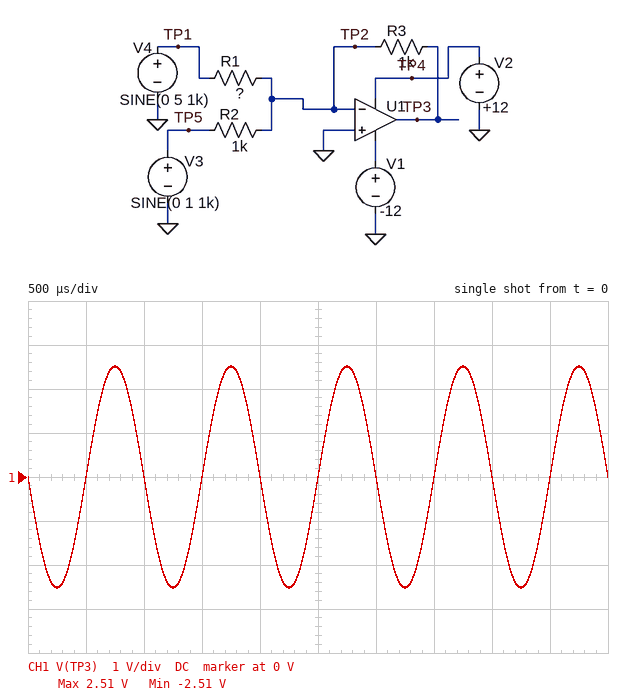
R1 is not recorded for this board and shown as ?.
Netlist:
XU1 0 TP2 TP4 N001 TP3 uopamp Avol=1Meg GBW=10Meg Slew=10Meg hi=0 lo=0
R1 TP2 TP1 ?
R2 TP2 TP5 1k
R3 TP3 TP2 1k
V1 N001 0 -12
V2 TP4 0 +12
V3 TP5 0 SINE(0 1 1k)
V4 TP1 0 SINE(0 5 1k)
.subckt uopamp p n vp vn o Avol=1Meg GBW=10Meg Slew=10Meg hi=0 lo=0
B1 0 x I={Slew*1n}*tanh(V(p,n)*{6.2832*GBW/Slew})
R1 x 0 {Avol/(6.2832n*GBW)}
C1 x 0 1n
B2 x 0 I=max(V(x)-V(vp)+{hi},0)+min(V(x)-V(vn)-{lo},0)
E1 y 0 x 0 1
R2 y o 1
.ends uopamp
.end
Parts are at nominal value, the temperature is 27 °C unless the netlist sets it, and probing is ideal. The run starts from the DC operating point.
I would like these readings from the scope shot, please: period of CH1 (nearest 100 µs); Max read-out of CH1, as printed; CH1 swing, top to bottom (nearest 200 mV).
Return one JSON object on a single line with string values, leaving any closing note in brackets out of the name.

{"period of CH1": "1.0 ms", "Max read-out of CH1, as printed": "2.51 V", "CH1 swing, top to bottom": "5.0 V"}
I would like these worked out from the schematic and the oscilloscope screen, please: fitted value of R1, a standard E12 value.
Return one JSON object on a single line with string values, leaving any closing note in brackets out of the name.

{"fitted value of R1, a standard E12 value": "3.3 kΩ"}
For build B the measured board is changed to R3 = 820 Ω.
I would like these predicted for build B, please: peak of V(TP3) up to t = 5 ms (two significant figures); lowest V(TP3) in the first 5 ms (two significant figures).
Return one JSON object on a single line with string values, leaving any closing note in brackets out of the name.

{"peak of V(TP3) up to t = 5 ms": "2.1 V", "lowest V(TP3) in the first 5 ms": "-2.1 V"}
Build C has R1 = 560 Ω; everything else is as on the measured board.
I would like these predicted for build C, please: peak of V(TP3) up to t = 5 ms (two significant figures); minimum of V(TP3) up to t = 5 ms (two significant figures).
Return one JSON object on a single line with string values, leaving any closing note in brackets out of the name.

{"peak of V(TP3) up to t = 5 ms": "9.9 V", "minimum of V(TP3) up to t = 5 ms": "-9.9 V"}
